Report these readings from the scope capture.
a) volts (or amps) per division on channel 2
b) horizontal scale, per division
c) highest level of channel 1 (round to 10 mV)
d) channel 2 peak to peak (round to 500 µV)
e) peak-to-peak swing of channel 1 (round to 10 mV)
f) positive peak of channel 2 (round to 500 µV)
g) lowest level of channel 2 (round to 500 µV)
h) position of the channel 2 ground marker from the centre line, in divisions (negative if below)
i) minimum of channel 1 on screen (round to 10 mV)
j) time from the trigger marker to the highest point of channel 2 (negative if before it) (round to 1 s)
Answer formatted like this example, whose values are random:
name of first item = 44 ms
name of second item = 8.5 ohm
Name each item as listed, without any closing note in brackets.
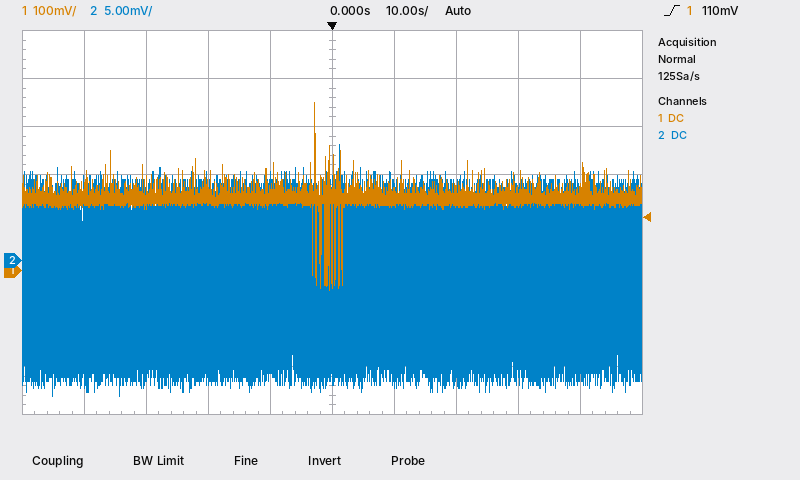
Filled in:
volts (or amps) per division on channel 2 = 5 mV
horizontal scale, per division = 10 s
highest level of channel 1 = 350 mV
channel 2 peak to peak = 26.0 mV
peak-to-peak swing of channel 1 = 390 mV
positive peak of channel 2 = 12.0 mV
lowest level of channel 2 = -14.0 mV
position of the channel 2 ground marker from the centre line, in divisions = -0.8 div
minimum of channel 1 on screen = -40 mV
time from the trigger marker to the highest point of channel 2 (negative if before it) = +1 s
